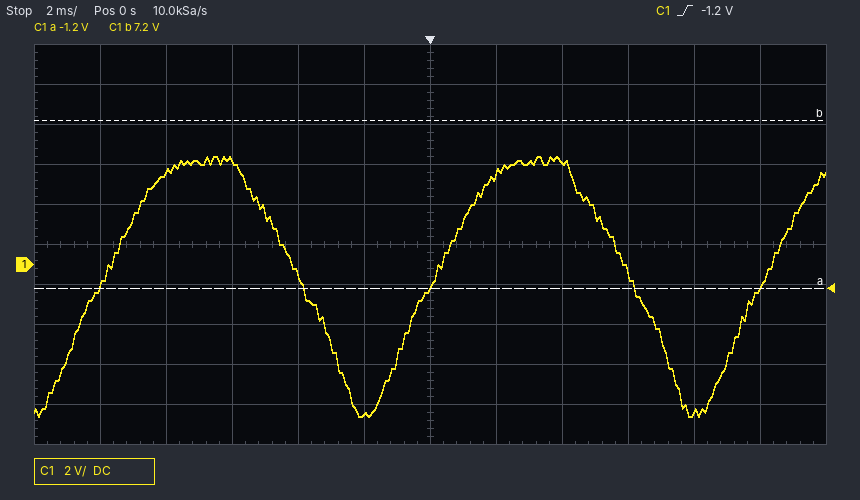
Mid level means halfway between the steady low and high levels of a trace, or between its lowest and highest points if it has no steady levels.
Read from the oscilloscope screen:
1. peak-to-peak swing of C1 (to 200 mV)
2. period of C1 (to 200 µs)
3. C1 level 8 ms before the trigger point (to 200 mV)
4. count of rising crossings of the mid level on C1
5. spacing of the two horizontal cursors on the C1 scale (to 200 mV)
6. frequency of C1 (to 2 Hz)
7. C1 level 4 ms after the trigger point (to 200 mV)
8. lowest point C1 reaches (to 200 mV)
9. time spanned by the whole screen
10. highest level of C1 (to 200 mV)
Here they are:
13.0 V
10.0 ms
4.6 V
3
8.4 V
100 Hz
5.2 V
-7.6 V
24 ms
5.4 V
